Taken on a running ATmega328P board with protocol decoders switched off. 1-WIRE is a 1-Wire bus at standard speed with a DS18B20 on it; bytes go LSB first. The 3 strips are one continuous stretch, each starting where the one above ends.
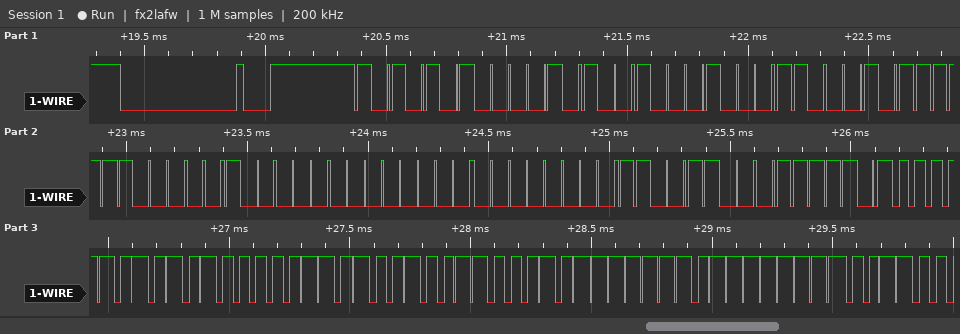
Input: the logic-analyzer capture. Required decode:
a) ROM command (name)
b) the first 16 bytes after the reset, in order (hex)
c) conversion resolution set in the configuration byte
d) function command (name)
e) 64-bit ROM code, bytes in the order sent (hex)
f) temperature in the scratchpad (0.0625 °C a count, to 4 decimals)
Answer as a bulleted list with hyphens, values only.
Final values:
- Match ROM
- 55 28 11 A3 1F 04 00 00 33 BE 50 05 4B 46 7F FF
- 12 bits
- Read Scratchpad
- 28 11 A3 1F 04 00 00 33
- 85.0000 °C
